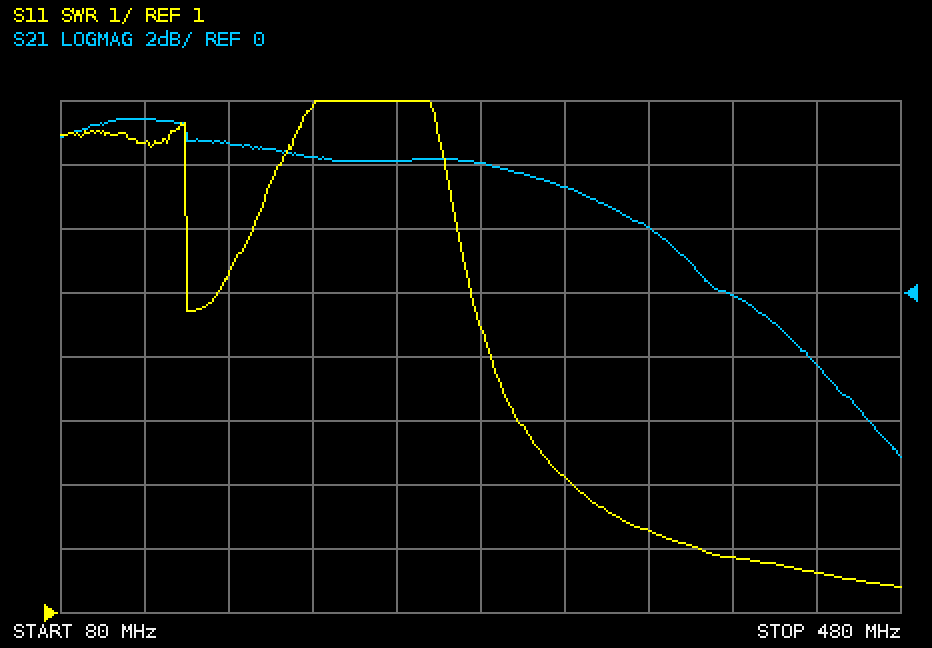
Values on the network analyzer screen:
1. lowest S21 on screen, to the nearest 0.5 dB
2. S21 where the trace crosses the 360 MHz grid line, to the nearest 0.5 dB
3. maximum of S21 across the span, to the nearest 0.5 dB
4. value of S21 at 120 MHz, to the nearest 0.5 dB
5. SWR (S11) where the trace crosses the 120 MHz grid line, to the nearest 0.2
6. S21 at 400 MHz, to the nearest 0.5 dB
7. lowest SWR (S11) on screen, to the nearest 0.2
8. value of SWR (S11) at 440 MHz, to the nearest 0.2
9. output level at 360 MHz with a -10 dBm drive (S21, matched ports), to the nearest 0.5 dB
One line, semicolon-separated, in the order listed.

-5.0 dB; 2.0 dB; 5.5 dB; 5.5 dB; 8.4; 0.0 dB; 1.4; 1.6; -8.0 dBm
